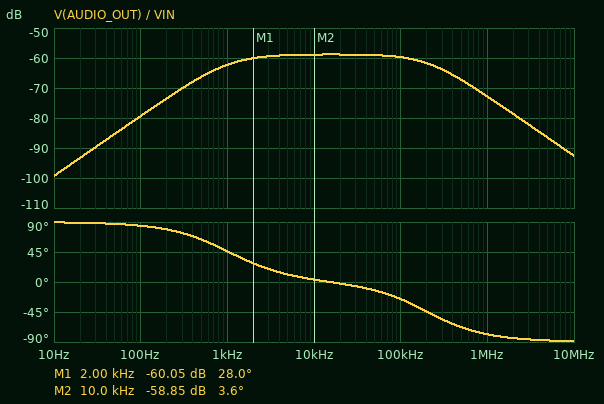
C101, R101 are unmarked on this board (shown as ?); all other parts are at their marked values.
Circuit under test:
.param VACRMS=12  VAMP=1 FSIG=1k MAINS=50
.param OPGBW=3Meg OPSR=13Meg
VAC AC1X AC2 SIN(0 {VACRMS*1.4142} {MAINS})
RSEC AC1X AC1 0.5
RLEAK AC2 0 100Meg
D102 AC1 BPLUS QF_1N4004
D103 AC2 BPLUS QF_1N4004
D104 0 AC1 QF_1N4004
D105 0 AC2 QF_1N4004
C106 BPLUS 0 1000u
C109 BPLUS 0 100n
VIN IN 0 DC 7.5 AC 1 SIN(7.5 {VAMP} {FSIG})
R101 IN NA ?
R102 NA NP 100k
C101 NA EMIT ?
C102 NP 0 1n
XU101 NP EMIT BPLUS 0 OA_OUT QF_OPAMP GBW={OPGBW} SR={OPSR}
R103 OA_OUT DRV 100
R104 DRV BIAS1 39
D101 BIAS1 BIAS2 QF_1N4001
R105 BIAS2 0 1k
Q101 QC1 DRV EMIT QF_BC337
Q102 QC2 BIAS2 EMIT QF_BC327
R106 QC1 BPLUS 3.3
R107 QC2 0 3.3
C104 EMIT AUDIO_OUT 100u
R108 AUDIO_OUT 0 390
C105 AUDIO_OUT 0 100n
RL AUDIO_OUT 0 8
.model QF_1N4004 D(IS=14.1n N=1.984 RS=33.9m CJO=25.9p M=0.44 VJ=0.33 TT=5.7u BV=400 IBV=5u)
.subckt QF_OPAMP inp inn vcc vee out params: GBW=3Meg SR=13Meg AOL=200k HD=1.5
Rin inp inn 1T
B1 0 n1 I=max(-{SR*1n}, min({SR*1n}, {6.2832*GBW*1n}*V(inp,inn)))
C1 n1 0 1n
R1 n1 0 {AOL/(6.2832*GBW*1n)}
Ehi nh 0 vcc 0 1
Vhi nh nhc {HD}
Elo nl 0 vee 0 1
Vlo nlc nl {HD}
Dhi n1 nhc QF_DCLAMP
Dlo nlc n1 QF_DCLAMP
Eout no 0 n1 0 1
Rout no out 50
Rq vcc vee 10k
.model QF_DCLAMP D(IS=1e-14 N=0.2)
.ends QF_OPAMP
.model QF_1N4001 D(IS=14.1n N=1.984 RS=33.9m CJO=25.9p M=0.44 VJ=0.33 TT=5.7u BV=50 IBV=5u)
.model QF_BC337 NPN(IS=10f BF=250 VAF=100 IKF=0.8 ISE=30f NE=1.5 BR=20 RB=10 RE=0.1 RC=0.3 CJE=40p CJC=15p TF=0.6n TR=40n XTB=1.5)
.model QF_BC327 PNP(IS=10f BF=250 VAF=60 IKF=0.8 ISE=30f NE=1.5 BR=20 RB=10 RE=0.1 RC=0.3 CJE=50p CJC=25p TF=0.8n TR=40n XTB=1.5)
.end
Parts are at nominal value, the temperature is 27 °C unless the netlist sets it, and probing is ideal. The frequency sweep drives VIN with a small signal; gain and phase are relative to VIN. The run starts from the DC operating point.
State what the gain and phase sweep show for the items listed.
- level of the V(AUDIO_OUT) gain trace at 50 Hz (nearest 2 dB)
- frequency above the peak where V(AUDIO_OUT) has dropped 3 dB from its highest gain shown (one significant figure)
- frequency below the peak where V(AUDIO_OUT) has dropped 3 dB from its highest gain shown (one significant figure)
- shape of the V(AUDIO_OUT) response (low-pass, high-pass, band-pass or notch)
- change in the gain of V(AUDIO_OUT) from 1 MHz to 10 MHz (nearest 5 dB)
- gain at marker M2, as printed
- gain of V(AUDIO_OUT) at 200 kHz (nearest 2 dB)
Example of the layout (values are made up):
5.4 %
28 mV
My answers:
-86 dB
200 kHz
1 kHz
band-pass
-20 dB
-58.85 dB
-62 dB
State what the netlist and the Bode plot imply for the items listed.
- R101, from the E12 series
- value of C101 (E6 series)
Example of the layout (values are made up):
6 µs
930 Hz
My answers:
6.8 kΩ
22 nF
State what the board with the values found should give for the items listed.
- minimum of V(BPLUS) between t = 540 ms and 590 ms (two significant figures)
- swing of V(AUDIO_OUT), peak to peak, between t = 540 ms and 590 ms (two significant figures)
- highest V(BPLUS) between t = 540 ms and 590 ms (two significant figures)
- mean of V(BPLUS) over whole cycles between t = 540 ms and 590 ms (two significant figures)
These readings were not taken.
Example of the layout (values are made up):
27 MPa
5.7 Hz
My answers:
15 V
2.5 V
15 V
15 V
